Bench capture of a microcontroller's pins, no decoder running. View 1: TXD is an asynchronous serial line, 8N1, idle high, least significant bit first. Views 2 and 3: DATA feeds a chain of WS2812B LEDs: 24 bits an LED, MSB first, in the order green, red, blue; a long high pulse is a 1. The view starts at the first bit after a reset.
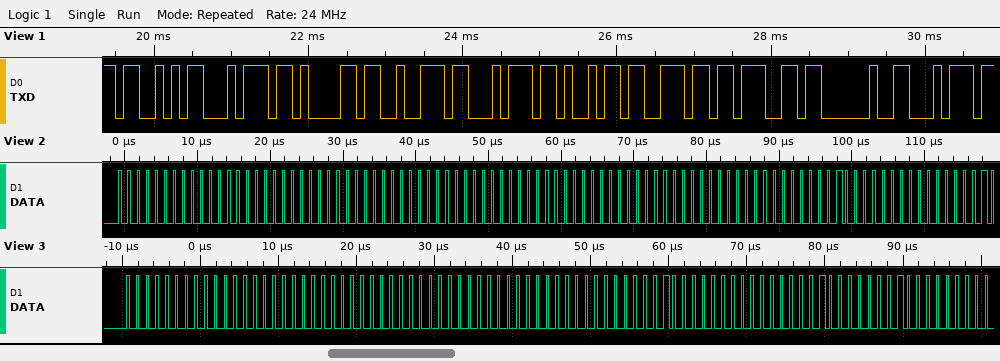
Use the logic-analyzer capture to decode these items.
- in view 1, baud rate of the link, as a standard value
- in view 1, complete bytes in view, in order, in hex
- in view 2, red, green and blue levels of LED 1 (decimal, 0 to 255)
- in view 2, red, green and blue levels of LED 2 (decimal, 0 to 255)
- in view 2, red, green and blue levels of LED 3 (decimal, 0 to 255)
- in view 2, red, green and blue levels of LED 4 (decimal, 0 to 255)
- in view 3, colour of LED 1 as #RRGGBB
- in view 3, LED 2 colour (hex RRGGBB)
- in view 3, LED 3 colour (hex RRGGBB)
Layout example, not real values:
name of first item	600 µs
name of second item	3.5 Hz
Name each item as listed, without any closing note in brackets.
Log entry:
in view 1, baud rate of the link, as a standard value	9600 baud
in view 1, complete bytes in view, in order, in hex	53 74 61 72 74 69 6E 67 20 74
in view 2, red, green and blue levels of LED 1	0, 0, 0
in view 2, red, green and blue levels of LED 2	0, 0, 0
in view 2, red, green and blue levels of LED 3	0, 0, 0
in view 2, red, green and blue levels of LED 4	0, 1, 1
in view 3, colour of LED 1 as #RRGGBB	#000000
in view 3, LED 2 colour	#000000
in view 3, LED 3 colour	#000101
